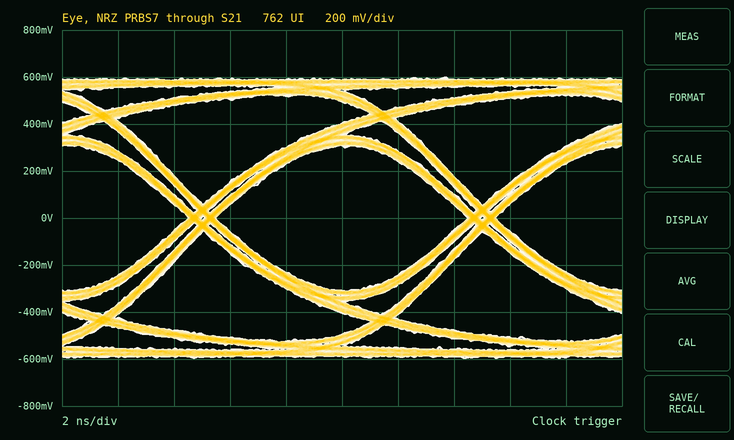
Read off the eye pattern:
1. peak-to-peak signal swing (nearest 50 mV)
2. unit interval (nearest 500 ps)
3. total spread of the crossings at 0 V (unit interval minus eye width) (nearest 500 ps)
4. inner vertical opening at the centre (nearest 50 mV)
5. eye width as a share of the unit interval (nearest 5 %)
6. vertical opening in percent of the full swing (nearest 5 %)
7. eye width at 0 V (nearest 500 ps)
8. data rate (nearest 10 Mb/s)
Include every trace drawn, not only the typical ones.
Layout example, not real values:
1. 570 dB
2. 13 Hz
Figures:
1. 1.20 V
2. 10.0 ns
3. 1.0 ns
4. 600 mV
5. 90 %
6. 50 %
7. 9.0 ns
8. 100 Mb/s
